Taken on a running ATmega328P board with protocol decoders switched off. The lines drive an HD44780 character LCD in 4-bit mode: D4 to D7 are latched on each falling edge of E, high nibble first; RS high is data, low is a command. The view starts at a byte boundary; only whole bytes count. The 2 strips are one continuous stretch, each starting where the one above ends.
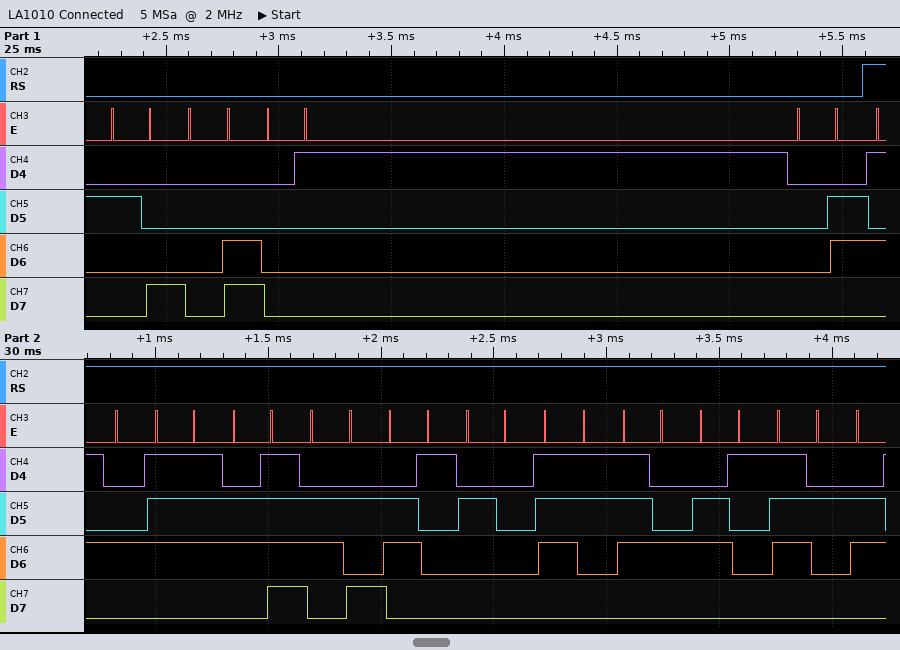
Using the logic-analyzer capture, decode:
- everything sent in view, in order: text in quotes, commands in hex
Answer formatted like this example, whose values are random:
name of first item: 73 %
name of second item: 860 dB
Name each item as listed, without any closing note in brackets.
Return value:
everything sent in view, in order: text in quotes, commands in hex: 0x28 0x0C 0x01 0x06 "Twoja star"
